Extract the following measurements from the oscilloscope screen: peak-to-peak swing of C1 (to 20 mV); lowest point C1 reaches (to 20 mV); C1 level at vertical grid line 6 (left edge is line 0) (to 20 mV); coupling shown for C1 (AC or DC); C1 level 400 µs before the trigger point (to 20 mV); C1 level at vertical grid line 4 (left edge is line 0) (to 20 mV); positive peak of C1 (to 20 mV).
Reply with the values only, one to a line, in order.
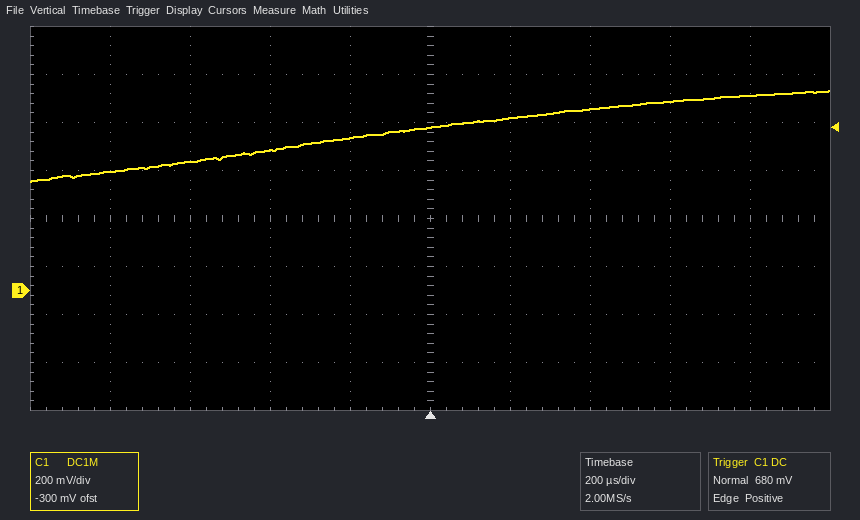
380 mV
460 mV
720 mV
DC
580 mV
640 mV
840 mV
